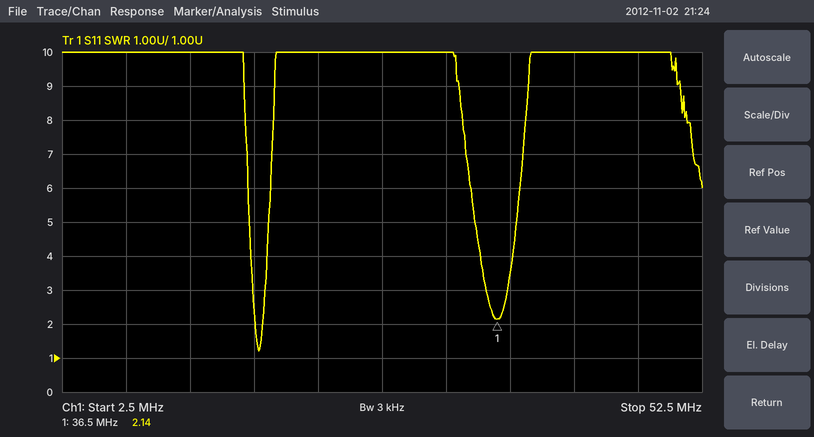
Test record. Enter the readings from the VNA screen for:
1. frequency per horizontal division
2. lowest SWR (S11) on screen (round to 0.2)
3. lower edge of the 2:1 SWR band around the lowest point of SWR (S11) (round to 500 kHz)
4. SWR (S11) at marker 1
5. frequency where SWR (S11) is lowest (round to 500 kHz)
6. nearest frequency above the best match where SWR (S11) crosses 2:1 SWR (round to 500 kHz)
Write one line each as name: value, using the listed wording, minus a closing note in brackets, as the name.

frequency per horizontal division: 5 MHz
lowest SWR (S11) on screen: 1.2
lower edge of the 2:1 SWR band around the lowest point of SWR (S11): 17.5 MHz
SWR (S11) at marker 1: 2.14
frequency where SWR (S11) is lowest: 18.0 MHz
nearest frequency above the best match where SWR (S11) crosses 2:1 SWR: 18.0 MHz
